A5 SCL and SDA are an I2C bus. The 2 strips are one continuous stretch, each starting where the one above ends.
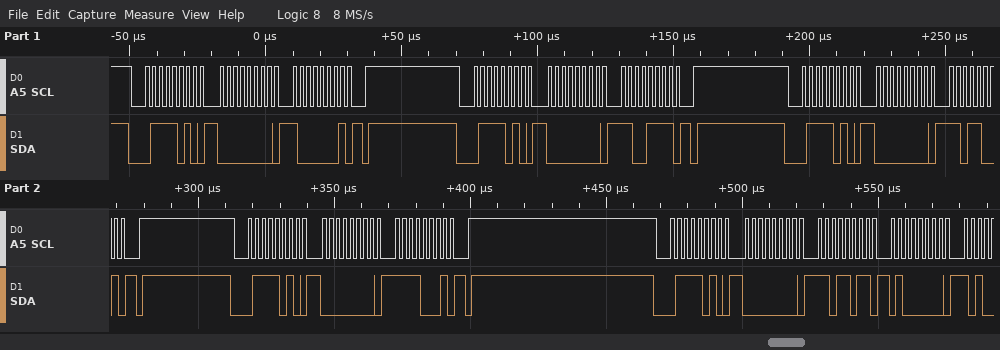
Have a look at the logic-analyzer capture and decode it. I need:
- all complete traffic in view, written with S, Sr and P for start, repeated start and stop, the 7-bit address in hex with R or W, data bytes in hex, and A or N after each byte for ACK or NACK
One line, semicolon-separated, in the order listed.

S 3DW A 00 A 81 A P S 3DW A 00 A CF A P S 3DW A 00 A D9 A P S 3DW A 00 A F1 A P S 3DW A 00 A DB A 40 A
